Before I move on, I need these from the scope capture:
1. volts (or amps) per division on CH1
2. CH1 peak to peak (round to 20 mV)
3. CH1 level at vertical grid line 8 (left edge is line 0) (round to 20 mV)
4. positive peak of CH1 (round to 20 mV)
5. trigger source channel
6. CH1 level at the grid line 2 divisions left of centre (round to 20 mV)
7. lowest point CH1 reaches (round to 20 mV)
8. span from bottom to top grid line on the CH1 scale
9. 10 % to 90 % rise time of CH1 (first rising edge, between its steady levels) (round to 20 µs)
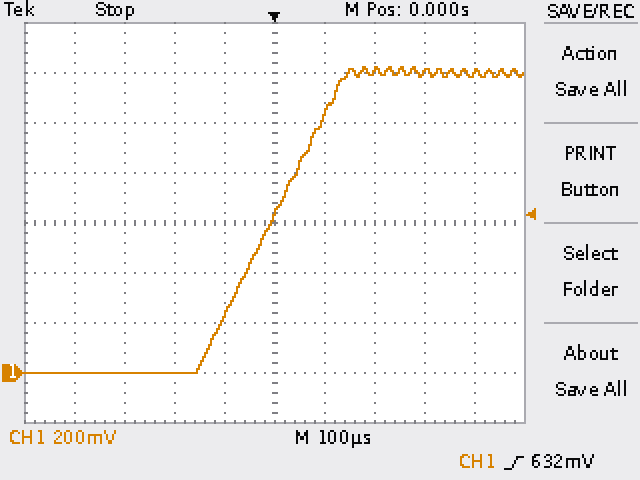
200 mV
1.22 V
1.20 V
1.22 V
CH1
0 mV
0 mV
1.6 V
240 µs
